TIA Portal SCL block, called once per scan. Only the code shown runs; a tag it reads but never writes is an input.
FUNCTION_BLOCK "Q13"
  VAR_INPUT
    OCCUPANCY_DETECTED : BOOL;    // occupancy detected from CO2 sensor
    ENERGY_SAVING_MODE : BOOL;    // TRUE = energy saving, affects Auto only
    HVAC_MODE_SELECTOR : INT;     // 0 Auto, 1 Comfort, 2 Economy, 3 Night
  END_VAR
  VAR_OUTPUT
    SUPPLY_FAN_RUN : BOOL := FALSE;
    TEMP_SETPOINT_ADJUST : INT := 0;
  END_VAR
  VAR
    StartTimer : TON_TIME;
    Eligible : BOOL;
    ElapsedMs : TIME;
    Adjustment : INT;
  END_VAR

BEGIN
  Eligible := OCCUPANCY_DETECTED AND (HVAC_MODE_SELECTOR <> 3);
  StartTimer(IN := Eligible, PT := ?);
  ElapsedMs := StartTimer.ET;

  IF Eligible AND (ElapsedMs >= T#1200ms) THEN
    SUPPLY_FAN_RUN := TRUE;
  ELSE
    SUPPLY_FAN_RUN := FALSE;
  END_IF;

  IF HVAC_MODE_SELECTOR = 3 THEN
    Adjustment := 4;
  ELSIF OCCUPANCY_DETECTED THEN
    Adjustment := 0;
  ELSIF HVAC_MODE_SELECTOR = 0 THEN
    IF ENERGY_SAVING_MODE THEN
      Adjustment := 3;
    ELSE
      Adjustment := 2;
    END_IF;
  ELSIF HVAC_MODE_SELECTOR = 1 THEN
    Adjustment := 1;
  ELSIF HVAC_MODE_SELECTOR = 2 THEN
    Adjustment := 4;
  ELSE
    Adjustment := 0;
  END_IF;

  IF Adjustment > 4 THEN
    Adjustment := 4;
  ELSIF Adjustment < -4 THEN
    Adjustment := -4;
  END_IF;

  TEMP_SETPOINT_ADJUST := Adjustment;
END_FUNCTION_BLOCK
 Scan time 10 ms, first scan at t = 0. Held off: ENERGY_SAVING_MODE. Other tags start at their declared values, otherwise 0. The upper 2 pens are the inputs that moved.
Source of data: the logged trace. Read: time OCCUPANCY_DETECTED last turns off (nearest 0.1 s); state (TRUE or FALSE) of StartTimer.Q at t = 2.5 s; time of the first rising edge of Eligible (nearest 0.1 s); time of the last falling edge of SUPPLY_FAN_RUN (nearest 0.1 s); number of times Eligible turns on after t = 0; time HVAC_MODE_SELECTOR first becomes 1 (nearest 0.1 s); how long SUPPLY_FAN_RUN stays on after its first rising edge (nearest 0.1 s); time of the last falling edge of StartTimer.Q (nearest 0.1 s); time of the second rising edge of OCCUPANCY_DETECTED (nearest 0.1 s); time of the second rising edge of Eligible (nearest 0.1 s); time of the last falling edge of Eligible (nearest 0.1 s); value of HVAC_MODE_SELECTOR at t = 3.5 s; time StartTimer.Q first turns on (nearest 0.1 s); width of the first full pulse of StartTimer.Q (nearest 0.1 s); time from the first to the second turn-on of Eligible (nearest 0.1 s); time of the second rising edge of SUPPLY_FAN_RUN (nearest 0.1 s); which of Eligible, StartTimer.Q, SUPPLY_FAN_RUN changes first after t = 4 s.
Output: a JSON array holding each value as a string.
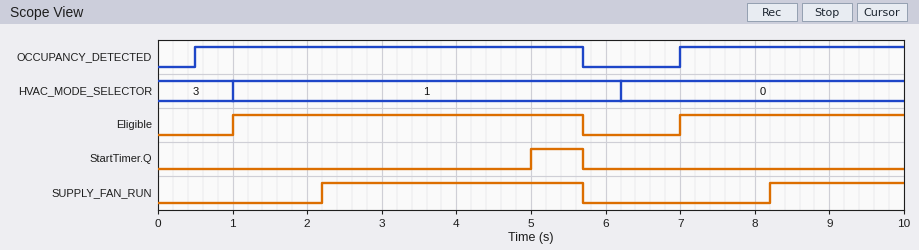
["5.7 s", "FALSE", "1.0 s", "5.7 s", "2", "1.0 s", "3.5 s", "5.7 s", "7.0 s", "7.0 s", "5.7 s", "1", "5.0 s", "0.7 s", "6.0 s", "8.2 s", "StartTimer.Q"]
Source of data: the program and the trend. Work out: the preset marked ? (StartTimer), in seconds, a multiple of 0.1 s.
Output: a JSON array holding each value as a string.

["4.0 s"]
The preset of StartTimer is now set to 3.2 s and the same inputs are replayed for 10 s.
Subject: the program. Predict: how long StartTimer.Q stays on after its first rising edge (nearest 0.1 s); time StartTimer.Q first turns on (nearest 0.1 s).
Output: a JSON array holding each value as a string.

["1.5 s", "4.2 s"]
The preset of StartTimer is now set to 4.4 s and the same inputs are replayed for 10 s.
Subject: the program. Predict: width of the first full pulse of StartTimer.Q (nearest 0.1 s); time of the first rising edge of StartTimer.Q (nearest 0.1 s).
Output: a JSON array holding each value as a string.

["0.3 s", "5.4 s"]
